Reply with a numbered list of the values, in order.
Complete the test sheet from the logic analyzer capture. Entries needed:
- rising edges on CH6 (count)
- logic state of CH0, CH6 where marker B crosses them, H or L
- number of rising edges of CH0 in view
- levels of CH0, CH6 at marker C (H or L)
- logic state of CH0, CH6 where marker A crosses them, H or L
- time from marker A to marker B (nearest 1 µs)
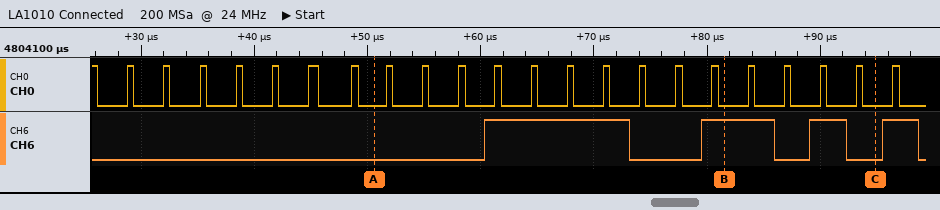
1. 4
2. CH0=L, CH6=H
3. 22
4. CH0=L, CH6=L
5. CH0=L, CH6=L
6. 31 µs
